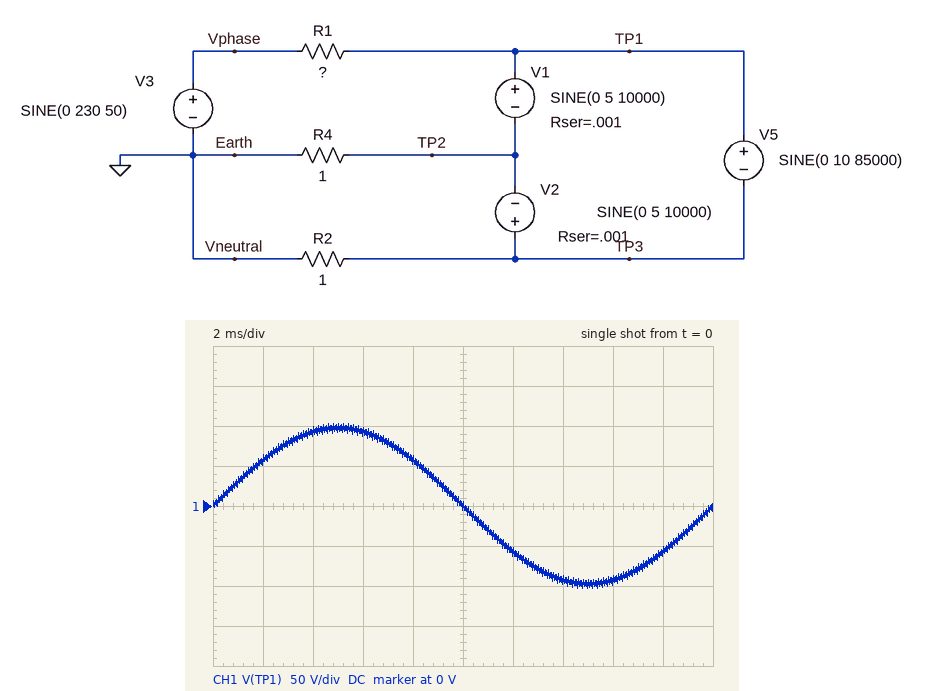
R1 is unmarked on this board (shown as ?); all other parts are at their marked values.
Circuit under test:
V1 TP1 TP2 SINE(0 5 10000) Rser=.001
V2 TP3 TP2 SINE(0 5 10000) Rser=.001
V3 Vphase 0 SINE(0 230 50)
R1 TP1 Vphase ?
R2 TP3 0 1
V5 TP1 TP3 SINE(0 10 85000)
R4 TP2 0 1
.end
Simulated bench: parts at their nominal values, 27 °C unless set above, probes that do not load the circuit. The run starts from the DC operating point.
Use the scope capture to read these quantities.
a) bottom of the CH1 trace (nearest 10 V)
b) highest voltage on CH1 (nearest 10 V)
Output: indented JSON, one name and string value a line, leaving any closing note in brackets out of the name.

{
  "bottom of the CH1 trace": "-100 V",
  "highest voltage on CH1": "100 V"
}
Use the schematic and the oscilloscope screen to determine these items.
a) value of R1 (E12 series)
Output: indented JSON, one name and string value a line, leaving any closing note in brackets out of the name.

{
  "value of R1": "0.68 Ω"
}
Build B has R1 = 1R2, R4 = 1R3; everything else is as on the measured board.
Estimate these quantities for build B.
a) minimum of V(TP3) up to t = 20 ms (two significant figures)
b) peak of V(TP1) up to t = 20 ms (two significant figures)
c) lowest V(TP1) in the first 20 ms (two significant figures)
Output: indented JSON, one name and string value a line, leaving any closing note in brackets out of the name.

{
  "minimum of V(TP3) up to t = 20 ms": "-79 V",
  "peak of V(TP1) up to t = 20 ms": "80 V",
  "lowest V(TP1) in the first 20 ms": "-80 V"
}
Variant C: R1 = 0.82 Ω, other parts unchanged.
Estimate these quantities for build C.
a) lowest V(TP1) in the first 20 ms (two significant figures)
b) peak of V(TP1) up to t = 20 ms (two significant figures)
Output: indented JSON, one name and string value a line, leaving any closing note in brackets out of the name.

{
  "lowest V(TP1) in the first 20 ms": "-93 V",
  "peak of V(TP1) up to t = 20 ms": "93 V"
}
